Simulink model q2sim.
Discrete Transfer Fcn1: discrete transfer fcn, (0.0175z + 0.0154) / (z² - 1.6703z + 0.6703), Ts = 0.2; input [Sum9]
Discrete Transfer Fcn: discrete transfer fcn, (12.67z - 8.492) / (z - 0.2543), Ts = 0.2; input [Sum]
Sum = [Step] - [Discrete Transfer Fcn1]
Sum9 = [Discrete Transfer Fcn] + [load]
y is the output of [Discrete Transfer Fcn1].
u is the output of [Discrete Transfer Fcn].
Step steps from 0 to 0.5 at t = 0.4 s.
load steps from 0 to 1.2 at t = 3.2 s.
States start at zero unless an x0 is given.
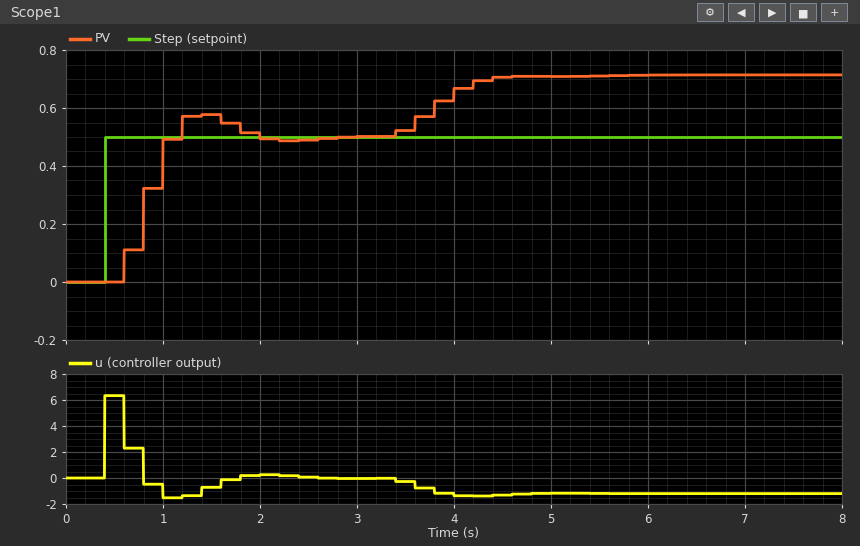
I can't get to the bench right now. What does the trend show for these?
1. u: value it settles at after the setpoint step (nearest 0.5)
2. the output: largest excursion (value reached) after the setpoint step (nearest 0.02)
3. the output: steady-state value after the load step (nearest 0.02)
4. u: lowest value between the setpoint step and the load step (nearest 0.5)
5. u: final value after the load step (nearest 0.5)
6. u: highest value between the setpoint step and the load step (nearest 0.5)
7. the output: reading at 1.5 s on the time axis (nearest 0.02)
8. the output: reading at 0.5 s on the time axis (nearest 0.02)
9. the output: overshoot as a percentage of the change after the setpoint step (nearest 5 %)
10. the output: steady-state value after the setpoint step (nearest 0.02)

0.0
0.58
0.72
-1.5
-1.0
6.5
0.58
0.00
15 %
0.50
